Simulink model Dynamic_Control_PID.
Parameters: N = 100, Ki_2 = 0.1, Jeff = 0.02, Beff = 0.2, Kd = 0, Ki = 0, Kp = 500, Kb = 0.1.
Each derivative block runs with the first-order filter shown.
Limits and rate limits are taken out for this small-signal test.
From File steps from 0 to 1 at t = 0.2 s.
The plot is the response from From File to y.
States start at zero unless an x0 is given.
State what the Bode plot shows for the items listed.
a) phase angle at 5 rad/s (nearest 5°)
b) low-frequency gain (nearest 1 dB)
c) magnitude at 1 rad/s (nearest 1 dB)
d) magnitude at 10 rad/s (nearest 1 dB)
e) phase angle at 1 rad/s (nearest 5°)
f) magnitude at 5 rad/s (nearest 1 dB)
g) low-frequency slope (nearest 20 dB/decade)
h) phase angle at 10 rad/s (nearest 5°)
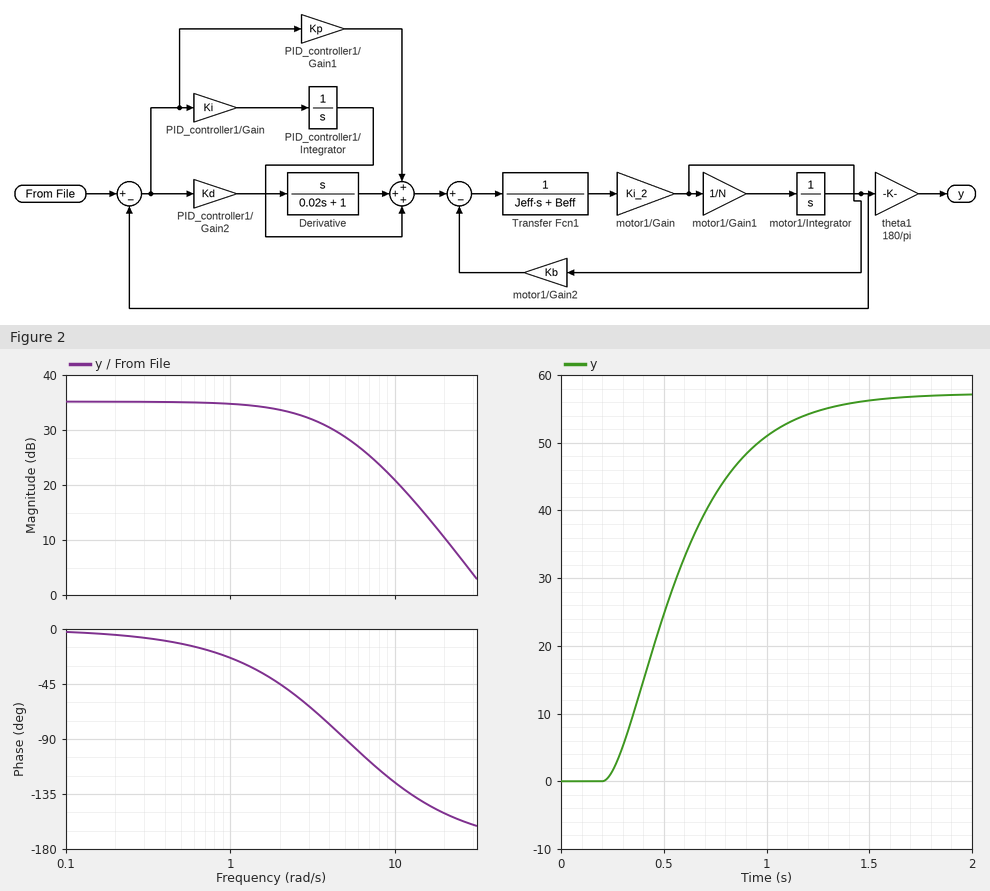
-90°
35 dB
35 dB
21 dB
-25°
29 dB
0 dB/decade
-125°
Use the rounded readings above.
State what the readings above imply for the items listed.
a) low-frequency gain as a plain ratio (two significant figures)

56
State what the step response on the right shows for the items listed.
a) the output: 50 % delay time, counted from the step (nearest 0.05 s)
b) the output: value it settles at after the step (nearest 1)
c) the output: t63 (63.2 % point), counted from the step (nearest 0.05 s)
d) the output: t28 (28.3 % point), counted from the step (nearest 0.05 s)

0.35 s
57
0.45 s
0.20 s
